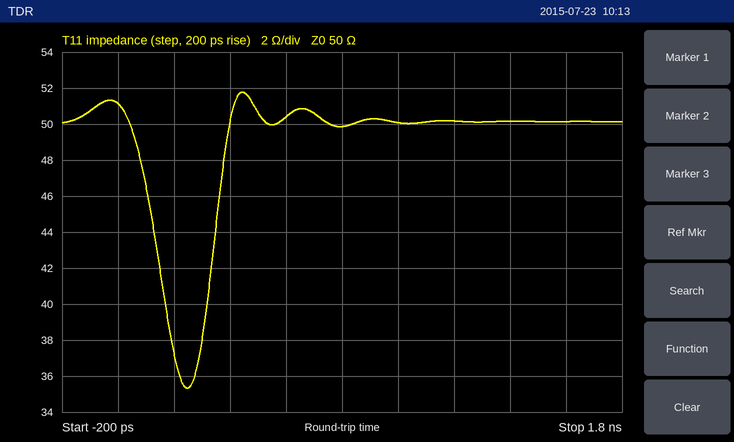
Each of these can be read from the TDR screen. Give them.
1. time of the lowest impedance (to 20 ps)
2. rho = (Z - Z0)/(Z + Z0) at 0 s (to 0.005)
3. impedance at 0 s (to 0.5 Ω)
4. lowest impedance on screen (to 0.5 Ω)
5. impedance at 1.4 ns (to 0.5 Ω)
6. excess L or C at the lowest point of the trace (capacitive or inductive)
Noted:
240 ps
+0.010
51.0 Ω
35.5 Ω
50.0 Ω
capacitive
